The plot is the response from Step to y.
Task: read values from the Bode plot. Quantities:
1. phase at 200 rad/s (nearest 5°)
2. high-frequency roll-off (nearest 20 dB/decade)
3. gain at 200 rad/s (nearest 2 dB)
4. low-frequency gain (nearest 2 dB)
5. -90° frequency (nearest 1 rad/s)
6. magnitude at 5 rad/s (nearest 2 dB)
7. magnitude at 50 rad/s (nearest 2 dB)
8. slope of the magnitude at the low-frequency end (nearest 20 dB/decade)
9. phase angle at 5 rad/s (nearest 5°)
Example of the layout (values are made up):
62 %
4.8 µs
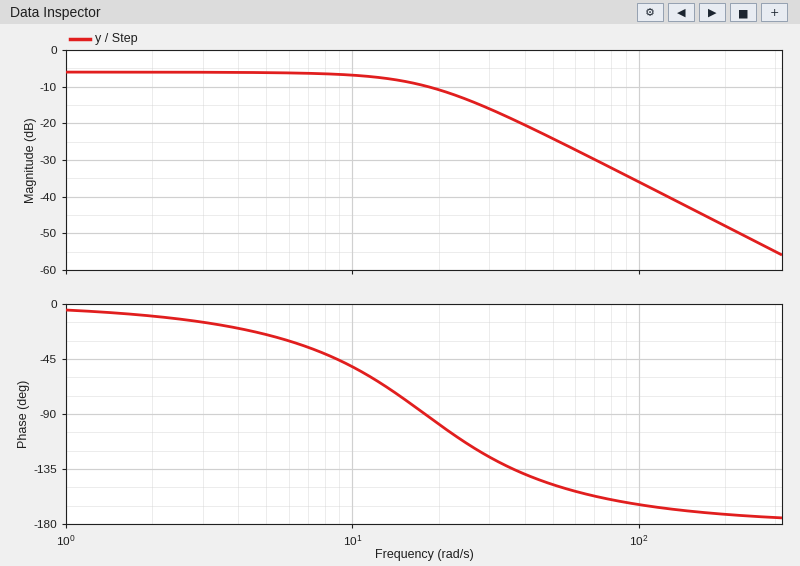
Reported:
-170°
-40 dB/decade
-48 dB
-6 dB
18 rad/s
-6 dB
-24 dB
0 dB/decade
-25°
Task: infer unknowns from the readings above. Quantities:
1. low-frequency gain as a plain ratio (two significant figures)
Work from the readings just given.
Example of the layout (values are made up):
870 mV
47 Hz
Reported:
0.50
